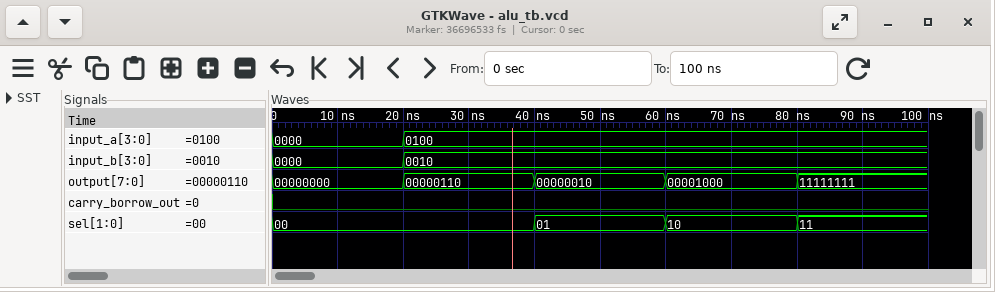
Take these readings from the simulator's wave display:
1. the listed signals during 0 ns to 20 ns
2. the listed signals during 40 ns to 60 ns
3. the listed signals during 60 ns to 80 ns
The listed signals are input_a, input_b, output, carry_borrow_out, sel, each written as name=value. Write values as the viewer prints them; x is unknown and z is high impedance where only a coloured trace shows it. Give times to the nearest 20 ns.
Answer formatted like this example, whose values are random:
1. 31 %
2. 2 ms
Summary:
1. input_a=0000, input_b=0000, output=00000000, carry_borrow_out=0, sel=00
2. input_a=0100, input_b=0010, output=00000010, carry_borrow_out=0, sel=01
3. input_a=0100, input_b=0010, output=00001000, carry_borrow_out=0, sel=10
